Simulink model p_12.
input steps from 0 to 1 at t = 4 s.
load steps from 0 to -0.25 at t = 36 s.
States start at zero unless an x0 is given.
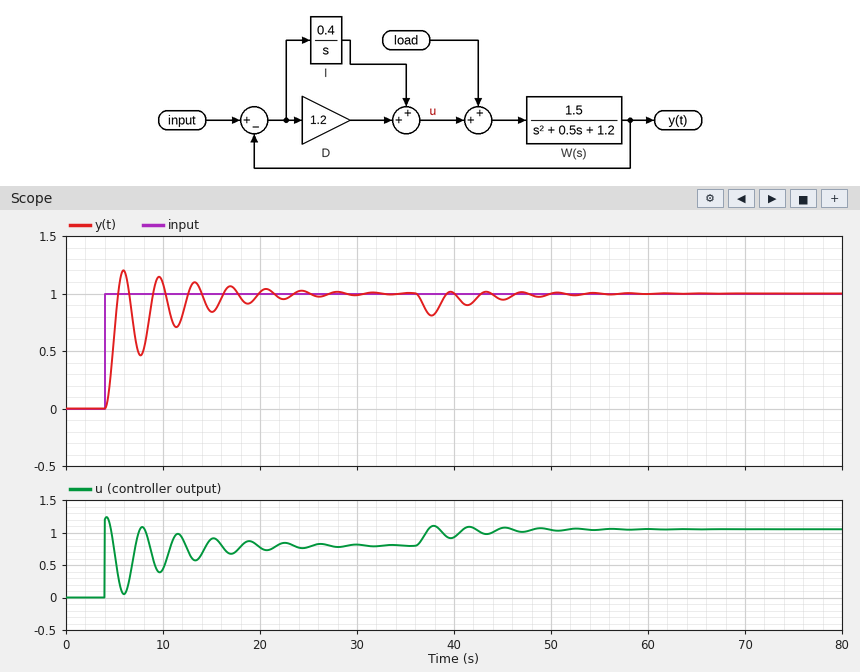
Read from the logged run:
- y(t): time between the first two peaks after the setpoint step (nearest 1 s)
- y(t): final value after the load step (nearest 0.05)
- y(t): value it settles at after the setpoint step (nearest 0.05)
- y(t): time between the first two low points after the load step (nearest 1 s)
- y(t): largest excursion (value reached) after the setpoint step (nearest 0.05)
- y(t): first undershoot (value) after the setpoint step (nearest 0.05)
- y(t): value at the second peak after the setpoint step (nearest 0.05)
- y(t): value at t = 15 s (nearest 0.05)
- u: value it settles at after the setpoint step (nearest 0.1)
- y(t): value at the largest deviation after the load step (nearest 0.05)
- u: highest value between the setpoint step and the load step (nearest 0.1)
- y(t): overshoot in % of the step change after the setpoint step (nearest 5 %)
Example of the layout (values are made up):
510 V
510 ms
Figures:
4 s
1.00
1.00
4 s
1.20
0.45
1.15
0.85
0.8
0.80
1.2
20 %
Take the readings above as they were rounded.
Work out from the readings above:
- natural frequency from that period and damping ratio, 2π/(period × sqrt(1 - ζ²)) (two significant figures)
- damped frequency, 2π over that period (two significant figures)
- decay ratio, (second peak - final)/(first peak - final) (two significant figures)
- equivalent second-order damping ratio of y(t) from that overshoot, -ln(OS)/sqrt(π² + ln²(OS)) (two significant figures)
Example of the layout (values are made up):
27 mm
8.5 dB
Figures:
1.8 rad/s
1.6 rad/s
0.75
0.46
